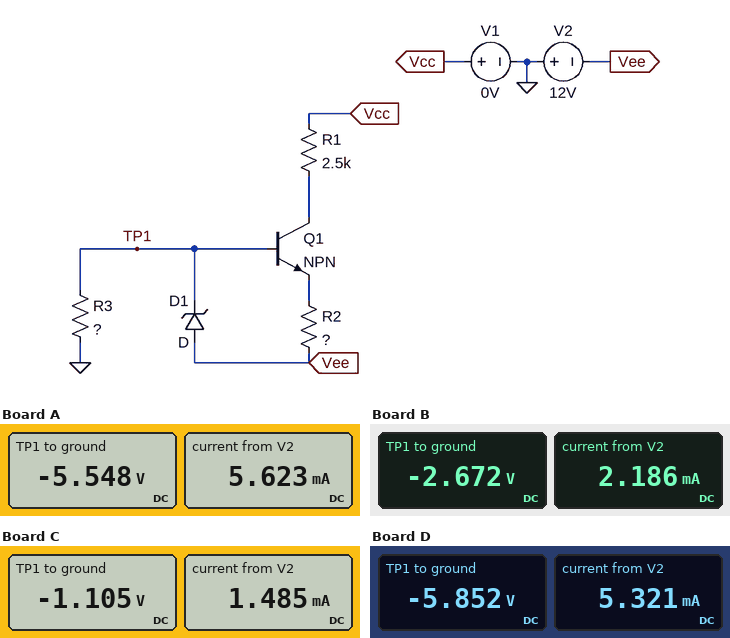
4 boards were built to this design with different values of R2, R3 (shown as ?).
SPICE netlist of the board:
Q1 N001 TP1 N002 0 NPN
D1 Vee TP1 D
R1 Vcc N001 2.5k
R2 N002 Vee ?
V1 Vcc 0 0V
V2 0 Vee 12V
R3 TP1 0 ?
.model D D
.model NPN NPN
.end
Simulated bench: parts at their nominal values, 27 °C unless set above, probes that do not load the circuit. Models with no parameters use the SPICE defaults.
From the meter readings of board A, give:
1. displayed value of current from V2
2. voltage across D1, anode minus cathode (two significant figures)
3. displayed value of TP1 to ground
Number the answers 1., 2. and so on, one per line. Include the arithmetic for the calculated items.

1. 5.623 mA
2. -12 V - (-5.548 V) = -6.5 V
3. -5.548 V
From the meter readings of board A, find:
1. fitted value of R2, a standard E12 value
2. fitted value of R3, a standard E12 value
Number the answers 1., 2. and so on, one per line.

1. 1 kΩ
2. 1.8 kΩ
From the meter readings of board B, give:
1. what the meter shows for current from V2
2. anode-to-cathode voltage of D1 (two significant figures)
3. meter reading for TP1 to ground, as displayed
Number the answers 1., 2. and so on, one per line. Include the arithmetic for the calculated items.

1. 2.186 mA
2. -12 V - (-2.672 V) = -9.3 V
3. -2.672 V
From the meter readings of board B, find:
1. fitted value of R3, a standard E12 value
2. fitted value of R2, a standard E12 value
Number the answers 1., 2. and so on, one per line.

1. 3.3 kΩ
2. 3.9 kΩ
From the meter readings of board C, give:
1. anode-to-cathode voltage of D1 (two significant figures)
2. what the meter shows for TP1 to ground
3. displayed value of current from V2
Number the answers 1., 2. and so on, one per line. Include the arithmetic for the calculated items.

1. -12 V - (-1.105 V) = -11 V
2. -1.105 V
3. 1.485 mA
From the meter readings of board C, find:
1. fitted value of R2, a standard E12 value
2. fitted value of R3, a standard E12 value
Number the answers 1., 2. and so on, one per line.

1. 6.8 kΩ
2. 1.5 kΩ
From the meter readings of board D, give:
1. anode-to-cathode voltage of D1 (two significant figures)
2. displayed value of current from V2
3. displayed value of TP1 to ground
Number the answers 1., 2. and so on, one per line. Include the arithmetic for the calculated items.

1. -12 V - (-5.852 V) = -6.1 V
2. 5.321 mA
3. -5.852 V
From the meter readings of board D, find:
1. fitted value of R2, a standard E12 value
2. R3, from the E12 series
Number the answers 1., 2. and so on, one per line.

1. 1 kΩ
2. 2.2 kΩ
